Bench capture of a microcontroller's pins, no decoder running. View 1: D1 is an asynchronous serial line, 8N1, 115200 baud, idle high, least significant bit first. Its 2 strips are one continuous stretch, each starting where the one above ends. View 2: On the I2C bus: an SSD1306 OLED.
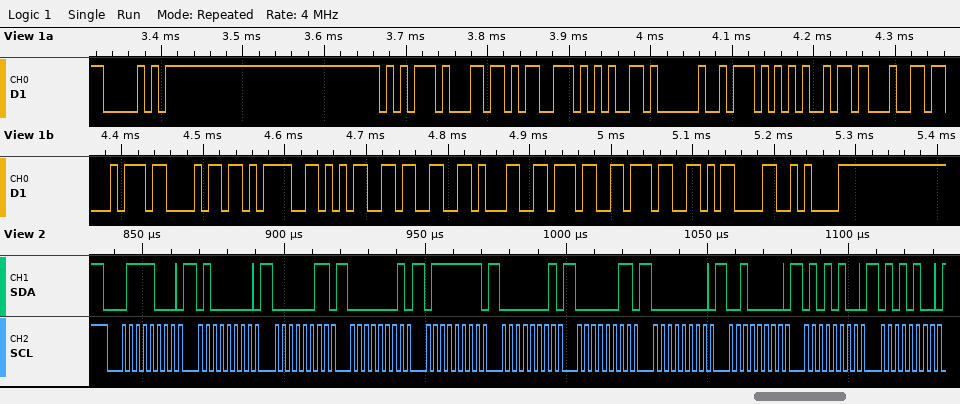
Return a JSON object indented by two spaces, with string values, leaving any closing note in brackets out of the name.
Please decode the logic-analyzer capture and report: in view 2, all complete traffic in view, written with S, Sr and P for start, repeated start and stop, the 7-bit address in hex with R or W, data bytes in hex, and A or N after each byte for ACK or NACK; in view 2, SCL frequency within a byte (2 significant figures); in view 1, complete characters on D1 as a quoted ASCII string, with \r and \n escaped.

{
  "in view 2, all complete traffic in view, written with S, Sr and P for start, repeated start and stop, the 7-bit address in hex with R or W, data bytes in hex, and A or N after each byte for ACK or NACK": "S 3CW A 40 A 03 A 01 A 7F A 01 A 03 A 00 A 20 A 54 A 54 A",
  "in view 2, SCL frequency within a byte": "400 kHz",
  "in view 1, complete characters on D1 as a quoted ASCII string, with \\r and \\n escaped": "\"Pulse Width=53177\\r\\n\""
}
